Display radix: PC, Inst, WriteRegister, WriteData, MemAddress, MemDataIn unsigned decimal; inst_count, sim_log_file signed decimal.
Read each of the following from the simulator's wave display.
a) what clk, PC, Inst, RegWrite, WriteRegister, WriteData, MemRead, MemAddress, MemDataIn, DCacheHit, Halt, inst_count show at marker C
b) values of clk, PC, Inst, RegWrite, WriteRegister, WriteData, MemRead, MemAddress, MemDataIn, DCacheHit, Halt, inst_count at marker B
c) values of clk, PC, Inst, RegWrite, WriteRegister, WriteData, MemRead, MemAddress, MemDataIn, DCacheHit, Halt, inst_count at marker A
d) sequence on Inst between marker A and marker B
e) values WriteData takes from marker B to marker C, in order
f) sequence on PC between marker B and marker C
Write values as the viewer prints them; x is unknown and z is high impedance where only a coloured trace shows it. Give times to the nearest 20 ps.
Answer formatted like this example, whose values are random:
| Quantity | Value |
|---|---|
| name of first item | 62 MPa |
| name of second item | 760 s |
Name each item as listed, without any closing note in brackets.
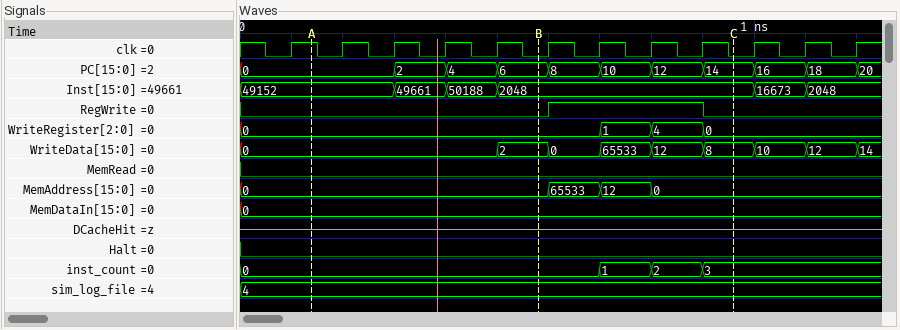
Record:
| Quantity | Value |
|---|---|
| what clk, PC, Inst, RegWrite, WriteRegister, WriteData, MemRead, MemAddress, MemDataIn, DCacheHit, Halt, inst_count show at marker C | clk=0, PC=14, Inst=2048, RegWrite=0, WriteRegister=0, WriteData=8, MemRead=0, MemAddress=0, MemDataIn=0, DCacheHit=z, Halt=0, inst_count=3 |
| values of clk, PC, Inst, RegWrite, WriteRegister, WriteData, MemRead, MemAddress, MemDataIn, DCacheHit, Halt, inst_count at marker B | clk=0, PC=6, Inst=2048, RegWrite=0, WriteRegister=0, WriteData=2, MemRead=0, MemAddress=0, MemDataIn=0, DCacheHit=z, Halt=0, inst_count=0 |
| values of clk, PC, Inst, RegWrite, WriteRegister, WriteData, MemRead, MemAddress, MemDataIn, DCacheHit, Halt, inst_count at marker A | clk=1, PC=0, Inst=49152, RegWrite=0, WriteRegister=0, WriteData=0, MemRead=0, MemAddress=0, MemDataIn=0, DCacheHit=z, Halt=0, inst_count=0 |
| sequence on Inst between marker A and marker B | 49152, 49661, 50188, 2048 |
| values WriteData takes from marker B to marker C, in order | 2, 0, 65533, 12, 8 |
| sequence on PC between marker B and marker C | 6, 8, 10, 12, 14 |
